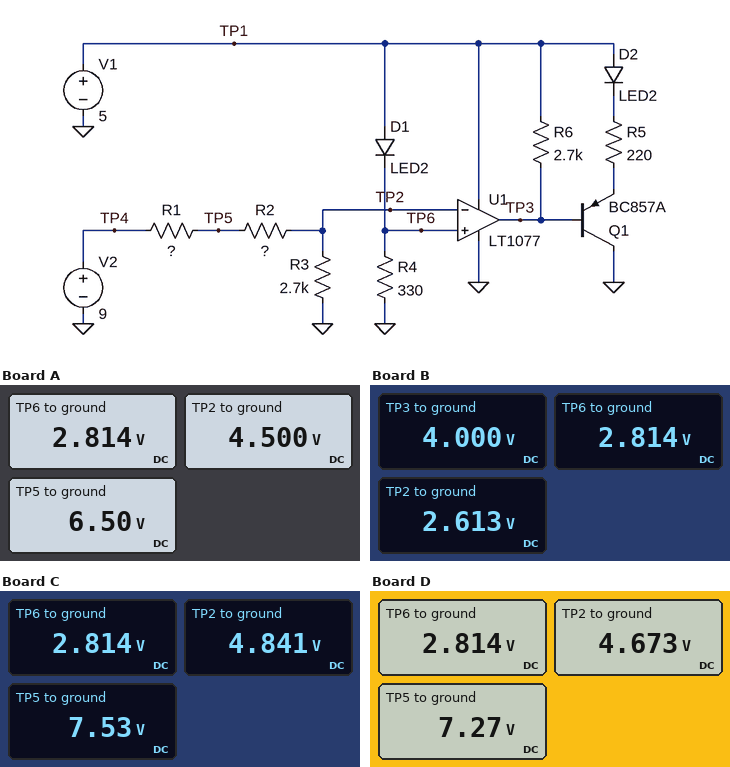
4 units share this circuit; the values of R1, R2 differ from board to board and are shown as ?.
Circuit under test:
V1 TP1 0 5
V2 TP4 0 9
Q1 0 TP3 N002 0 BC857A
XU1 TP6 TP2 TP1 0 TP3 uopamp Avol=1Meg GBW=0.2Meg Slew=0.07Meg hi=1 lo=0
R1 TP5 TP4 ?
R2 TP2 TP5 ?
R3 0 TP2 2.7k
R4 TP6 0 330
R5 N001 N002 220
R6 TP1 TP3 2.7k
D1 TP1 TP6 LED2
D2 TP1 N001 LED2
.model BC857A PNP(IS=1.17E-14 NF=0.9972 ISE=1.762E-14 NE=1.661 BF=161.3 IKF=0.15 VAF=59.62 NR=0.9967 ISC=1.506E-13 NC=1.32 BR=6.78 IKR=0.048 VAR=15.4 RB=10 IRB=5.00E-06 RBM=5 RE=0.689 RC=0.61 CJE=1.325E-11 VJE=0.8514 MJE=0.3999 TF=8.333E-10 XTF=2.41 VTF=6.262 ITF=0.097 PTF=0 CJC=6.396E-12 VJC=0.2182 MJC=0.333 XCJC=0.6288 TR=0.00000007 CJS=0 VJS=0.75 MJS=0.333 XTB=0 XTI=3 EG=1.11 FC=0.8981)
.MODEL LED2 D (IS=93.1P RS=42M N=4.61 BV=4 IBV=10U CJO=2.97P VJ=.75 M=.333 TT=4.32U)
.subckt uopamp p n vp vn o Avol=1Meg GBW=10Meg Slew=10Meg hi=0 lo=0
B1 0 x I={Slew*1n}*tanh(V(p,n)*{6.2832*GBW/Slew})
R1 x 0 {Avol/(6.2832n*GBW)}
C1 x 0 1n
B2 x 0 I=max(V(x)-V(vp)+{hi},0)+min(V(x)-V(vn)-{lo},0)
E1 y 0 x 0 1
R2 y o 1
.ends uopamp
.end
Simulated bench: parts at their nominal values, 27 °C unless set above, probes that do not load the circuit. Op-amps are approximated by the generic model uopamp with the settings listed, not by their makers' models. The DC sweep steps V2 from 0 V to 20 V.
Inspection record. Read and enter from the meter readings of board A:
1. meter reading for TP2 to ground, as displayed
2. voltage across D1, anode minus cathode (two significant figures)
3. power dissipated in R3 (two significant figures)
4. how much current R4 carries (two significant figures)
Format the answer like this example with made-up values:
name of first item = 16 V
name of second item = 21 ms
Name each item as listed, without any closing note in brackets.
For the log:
meter reading for TP2 to ground, as displayed = 4.500 V
voltage across D1, anode minus cathode = 2.2 V
power dissipated in R3 = 7.5 mW
how much current R4 carries = 8.5 mA
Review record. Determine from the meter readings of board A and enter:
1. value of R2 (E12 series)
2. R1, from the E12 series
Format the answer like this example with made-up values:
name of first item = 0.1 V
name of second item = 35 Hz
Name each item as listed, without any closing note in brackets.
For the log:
value of R2 = 1.2 kΩ
R1, from the E12 series = 1.5 kΩ
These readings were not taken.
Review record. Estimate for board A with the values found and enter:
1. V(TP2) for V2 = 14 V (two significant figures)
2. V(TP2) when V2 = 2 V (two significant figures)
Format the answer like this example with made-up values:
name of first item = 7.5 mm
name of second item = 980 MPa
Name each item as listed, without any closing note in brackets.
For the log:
V(TP2) for V2 = 14 V = 7.0 V
V(TP2) when V2 = 2 V = 1.0 V
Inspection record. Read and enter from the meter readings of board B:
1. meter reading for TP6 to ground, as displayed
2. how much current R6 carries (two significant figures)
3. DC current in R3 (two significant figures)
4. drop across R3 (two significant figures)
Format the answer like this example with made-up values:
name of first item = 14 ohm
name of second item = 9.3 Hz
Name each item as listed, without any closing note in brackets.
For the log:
meter reading for TP6 to ground, as displayed = 2.814 V
how much current R6 carries = 370 µA
DC current in R3 = 970 µA
drop across R3 = 2.6 V
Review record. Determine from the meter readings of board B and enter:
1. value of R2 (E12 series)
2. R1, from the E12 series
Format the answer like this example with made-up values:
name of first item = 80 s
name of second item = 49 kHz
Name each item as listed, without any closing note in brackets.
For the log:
value of R2 = 5.6 kΩ
R1, from the E12 series = 1 kΩ
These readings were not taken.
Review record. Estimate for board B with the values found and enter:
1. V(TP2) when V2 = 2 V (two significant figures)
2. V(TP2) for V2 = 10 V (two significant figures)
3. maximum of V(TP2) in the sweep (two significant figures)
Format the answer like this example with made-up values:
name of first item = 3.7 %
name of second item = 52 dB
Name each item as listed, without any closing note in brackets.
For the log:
V(TP2) when V2 = 2 V = 580 mV
V(TP2) for V2 = 10 V = 2.9 V
maximum of V(TP2) in the sweep = 5.8 V
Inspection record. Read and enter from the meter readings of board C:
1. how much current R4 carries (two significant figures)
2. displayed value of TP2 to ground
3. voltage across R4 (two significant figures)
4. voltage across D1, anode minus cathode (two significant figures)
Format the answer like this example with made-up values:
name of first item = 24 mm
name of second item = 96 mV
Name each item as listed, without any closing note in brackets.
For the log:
how much current R4 carries = 8.5 mA
displayed value of TP2 to ground = 4.841 V
voltage across R4 = 2.8 V
voltage across D1, anode minus cathode = 2.2 V
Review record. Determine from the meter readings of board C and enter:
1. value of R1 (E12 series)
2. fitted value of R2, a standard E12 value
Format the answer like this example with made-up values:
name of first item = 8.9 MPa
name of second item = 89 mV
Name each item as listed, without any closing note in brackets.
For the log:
value of R1 = 820 Ω
fitted value of R2, a standard E12 value = 1.5 kΩ
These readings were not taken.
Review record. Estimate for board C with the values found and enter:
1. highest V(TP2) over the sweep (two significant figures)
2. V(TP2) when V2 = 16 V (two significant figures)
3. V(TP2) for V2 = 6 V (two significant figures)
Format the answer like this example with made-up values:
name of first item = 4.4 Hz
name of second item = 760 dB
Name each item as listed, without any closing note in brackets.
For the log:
highest V(TP2) over the sweep = 11 V
V(TP2) when V2 = 16 V = 8.6 V
V(TP2) for V2 = 6 V = 3.2 V
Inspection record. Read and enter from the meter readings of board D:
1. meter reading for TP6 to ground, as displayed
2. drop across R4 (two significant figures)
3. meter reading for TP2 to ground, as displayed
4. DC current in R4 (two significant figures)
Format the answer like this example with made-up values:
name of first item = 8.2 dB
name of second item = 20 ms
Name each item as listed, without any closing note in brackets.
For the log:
meter reading for TP6 to ground, as displayed = 2.814 V
drop across R4 = 2.8 V
meter reading for TP2 to ground, as displayed = 4.673 V
DC current in R4 = 8.5 mA
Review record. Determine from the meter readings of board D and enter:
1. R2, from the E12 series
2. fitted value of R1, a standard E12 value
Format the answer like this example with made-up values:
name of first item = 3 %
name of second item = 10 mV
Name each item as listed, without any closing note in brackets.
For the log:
R2, from the E12 series = 1.5 kΩ
fitted value of R1, a standard E12 value = 1 kΩ
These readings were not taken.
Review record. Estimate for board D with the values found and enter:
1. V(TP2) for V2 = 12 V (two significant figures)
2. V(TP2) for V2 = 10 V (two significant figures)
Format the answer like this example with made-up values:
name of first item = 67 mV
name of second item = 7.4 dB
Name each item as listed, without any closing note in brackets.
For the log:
V(TP2) for V2 = 12 V = 6.2 V
V(TP2) for V2 = 10 V = 5.2 V
